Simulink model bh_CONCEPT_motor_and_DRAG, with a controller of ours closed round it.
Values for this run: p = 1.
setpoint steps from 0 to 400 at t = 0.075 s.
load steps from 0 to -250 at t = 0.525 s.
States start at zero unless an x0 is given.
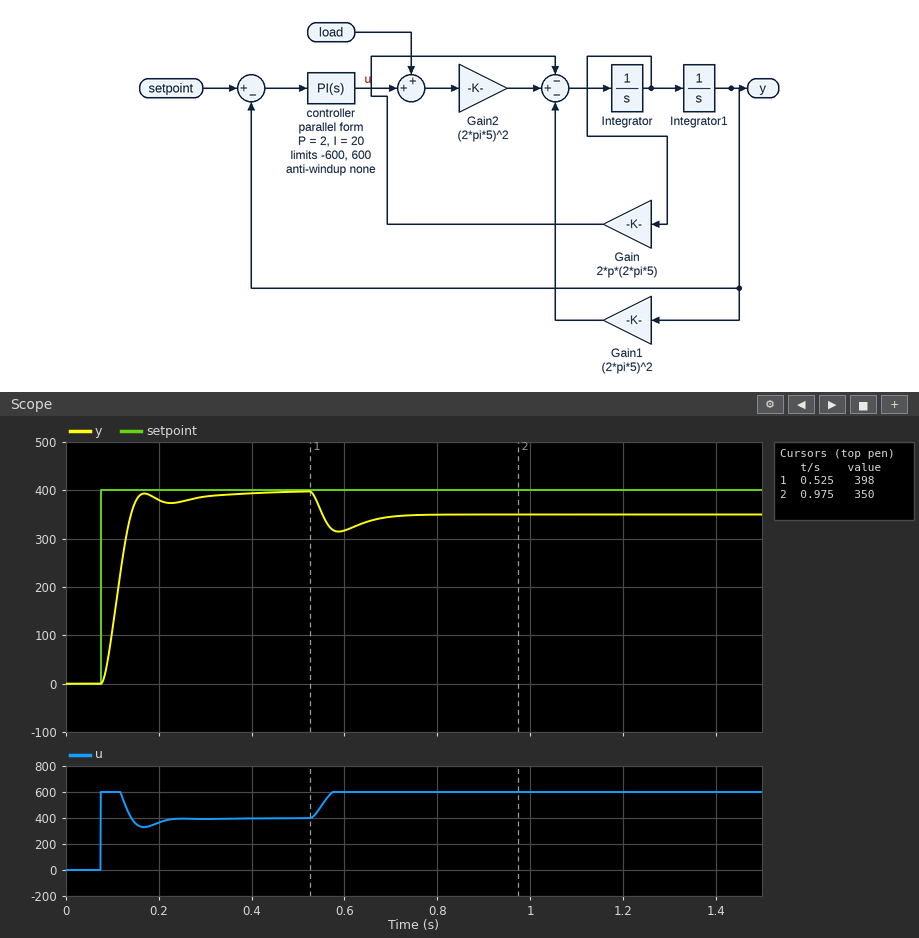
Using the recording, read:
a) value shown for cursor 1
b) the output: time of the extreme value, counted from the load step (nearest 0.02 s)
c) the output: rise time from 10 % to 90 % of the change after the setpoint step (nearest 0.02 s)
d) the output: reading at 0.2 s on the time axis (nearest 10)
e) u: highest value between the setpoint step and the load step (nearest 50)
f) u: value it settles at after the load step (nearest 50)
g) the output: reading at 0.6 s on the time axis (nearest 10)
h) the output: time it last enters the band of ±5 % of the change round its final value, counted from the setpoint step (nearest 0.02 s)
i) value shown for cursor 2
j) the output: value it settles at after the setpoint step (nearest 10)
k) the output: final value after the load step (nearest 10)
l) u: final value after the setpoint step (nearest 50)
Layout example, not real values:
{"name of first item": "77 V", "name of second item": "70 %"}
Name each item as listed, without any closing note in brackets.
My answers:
{"value shown for cursor 1": "398", "the output: time of the extreme value, counted from the load step": "0.06 s", "the output: rise time from 10 % to 90 % of the change after the setpoint step": "0.06 s", "the output: reading at 0.2 s on the time axis": "380", "u: highest value between the setpoint step and the load step": "600", "u: value it settles at after the load step": "600", "the output: reading at 0.6 s on the time axis": "320", "the output: time it last enters the band of ±5 % of the change round its final value, counted from the setpoint step": "0.18 s", "value shown for cursor 2": "350", "the output: value it settles at after the setpoint step": "400", "the output: final value after the load step": "350", "u: final value after the setpoint step": "400"}
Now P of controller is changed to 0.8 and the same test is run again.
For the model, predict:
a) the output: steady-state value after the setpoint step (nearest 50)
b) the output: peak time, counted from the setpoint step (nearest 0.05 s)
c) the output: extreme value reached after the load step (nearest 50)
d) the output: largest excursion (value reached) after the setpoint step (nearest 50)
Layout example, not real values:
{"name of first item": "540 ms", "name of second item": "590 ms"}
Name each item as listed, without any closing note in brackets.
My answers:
{"the output: steady-state value after the setpoint step": "400", "the output: peak time, counted from the setpoint step": "0.15 s", "the output: extreme value reached after the load step": "300", "the output: largest excursion (value reached) after the setpoint step": "400"}
